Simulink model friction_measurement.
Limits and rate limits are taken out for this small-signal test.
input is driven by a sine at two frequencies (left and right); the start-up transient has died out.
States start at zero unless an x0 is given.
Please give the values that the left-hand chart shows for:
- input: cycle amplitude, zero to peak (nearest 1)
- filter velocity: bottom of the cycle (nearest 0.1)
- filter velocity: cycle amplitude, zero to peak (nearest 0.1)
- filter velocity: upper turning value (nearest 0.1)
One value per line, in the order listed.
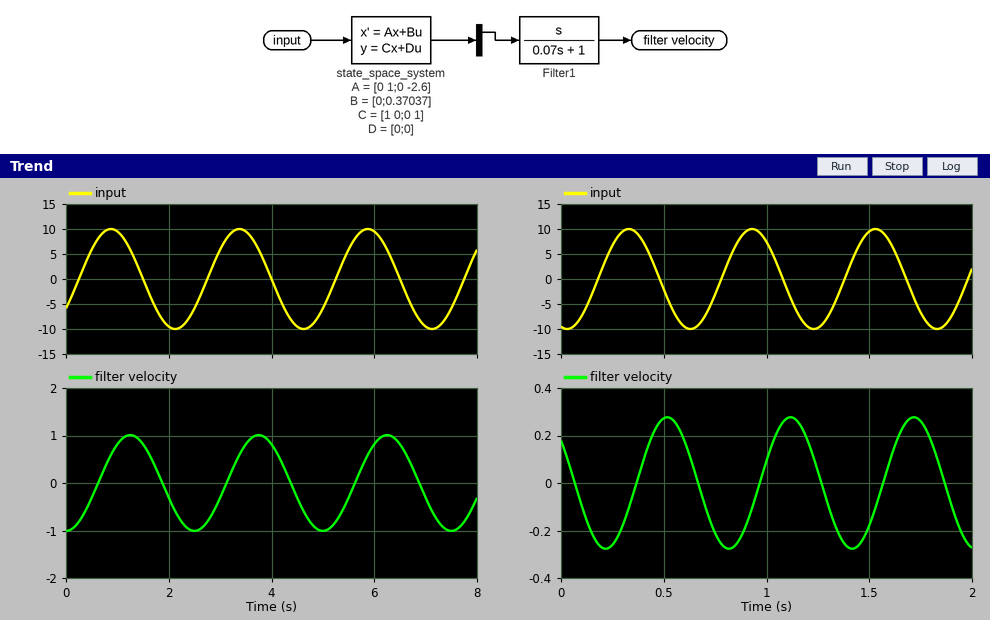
10
-1.0
1.0
1.0
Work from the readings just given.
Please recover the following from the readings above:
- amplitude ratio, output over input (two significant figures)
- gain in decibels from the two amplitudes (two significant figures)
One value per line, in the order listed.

0.10
-20 dB
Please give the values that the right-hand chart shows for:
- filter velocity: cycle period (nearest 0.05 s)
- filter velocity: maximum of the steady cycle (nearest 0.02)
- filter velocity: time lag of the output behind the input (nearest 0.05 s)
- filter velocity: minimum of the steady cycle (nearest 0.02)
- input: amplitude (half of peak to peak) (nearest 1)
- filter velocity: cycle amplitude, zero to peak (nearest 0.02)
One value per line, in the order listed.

0.60 s
0.28
0.20 s
-0.28
10
0.28
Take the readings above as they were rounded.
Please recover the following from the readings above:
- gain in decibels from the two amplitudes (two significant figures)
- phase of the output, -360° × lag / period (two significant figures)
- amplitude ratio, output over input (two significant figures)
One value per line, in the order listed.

-31 dB
-120°
0.028
